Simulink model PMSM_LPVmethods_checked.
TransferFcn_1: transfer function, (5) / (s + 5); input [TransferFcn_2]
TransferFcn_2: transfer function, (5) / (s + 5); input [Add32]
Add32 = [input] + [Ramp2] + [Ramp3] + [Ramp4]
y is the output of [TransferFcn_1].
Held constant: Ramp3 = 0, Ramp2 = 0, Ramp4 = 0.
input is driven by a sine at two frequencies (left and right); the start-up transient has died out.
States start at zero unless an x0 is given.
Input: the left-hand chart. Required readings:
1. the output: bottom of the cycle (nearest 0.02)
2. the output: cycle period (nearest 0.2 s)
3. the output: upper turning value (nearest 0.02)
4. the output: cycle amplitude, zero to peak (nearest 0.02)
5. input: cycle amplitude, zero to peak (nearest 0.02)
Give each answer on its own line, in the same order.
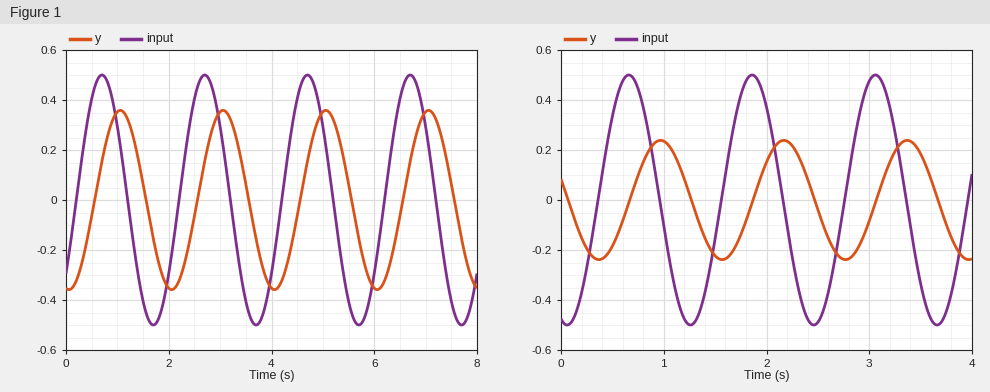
-0.36
2.0 s
0.36
0.36
0.50
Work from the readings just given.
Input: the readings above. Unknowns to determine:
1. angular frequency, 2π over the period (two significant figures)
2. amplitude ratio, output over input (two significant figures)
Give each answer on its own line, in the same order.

3.1 rad/s
0.72
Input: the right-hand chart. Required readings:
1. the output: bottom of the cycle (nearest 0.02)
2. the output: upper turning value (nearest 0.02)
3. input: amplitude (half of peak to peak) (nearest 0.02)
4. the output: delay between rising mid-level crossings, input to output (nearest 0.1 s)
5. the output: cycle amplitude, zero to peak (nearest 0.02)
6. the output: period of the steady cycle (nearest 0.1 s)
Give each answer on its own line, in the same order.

-0.24
0.24
0.50
0.3 s
0.24
1.2 s
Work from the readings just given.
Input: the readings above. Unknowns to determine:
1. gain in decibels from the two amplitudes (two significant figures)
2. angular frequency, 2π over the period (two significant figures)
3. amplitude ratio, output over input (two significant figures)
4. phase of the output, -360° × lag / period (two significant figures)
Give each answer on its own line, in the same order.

-6.4 dB
5.2 rad/s
0.48
-90°
